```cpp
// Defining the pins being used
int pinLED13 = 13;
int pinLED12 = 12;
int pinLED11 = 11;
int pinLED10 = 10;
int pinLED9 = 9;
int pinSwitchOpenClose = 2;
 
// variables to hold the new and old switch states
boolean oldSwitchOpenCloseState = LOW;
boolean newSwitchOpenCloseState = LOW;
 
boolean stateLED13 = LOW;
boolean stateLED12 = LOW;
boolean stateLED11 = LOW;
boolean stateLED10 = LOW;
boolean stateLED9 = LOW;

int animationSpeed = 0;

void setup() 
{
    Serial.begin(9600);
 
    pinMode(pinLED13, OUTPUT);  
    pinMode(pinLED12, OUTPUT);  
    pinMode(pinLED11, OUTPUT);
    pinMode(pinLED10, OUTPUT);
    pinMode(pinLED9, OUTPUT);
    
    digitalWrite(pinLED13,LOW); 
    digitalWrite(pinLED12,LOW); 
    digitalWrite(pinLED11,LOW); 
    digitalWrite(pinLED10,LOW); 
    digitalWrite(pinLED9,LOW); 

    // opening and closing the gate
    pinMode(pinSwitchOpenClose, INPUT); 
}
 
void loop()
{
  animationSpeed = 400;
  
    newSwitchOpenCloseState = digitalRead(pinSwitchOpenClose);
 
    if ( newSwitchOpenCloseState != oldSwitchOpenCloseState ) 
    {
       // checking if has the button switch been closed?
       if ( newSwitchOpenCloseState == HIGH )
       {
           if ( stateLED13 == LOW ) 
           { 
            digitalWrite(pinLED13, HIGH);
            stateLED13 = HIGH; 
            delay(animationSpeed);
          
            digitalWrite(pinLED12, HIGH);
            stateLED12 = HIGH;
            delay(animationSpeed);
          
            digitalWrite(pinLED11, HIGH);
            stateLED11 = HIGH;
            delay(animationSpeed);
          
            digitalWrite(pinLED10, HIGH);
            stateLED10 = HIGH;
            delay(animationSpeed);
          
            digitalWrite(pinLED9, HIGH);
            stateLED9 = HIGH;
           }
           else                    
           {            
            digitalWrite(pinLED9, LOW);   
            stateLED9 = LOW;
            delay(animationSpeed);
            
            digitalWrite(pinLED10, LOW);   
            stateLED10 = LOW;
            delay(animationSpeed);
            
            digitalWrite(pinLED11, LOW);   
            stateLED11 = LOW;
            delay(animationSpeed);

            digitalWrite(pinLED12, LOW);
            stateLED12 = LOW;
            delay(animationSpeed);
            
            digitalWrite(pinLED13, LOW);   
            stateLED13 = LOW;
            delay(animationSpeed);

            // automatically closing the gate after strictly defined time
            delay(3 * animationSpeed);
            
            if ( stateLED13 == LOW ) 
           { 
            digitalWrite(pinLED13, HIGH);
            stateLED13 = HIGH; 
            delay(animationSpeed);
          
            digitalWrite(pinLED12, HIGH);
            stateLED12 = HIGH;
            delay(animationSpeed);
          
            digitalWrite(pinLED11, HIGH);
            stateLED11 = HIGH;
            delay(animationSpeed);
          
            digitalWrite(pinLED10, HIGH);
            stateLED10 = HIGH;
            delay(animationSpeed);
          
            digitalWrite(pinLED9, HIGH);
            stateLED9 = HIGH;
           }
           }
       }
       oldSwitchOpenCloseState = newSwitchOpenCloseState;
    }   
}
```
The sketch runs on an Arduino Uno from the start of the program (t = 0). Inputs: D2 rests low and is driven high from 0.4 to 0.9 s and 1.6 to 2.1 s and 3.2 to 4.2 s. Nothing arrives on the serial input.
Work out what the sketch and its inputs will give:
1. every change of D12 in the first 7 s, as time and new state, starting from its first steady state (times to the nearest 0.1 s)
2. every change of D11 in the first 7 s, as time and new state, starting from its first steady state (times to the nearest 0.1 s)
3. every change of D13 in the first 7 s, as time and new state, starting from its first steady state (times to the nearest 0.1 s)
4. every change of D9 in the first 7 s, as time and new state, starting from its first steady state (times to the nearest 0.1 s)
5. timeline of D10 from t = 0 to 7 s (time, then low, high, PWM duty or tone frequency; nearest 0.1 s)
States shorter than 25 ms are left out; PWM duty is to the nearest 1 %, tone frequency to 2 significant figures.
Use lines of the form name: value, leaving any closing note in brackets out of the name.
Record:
every change of D12 in the first 7 s, as time and new state, starting from its first steady state: 0 s low; 0.8 s high; 4.4 s low; 6.8 s high
every change of D11 in the first 7 s, as time and new state, starting from its first steady state: 0 s low; 1.2 s high; 4 s low
every change of D13 in the first 7 s, as time and new state, starting from its first steady state: 0 s low; 0.4 s high; 4.8 s low; 6.4 s high
every change of D9 in the first 7 s, as time and new state, starting from its first steady state: 0 s low; 2 s high; 3.2 s low
timeline of D10 from t = 0 to 7 s: 0 s low; 1.6 s high; 3.6 s low
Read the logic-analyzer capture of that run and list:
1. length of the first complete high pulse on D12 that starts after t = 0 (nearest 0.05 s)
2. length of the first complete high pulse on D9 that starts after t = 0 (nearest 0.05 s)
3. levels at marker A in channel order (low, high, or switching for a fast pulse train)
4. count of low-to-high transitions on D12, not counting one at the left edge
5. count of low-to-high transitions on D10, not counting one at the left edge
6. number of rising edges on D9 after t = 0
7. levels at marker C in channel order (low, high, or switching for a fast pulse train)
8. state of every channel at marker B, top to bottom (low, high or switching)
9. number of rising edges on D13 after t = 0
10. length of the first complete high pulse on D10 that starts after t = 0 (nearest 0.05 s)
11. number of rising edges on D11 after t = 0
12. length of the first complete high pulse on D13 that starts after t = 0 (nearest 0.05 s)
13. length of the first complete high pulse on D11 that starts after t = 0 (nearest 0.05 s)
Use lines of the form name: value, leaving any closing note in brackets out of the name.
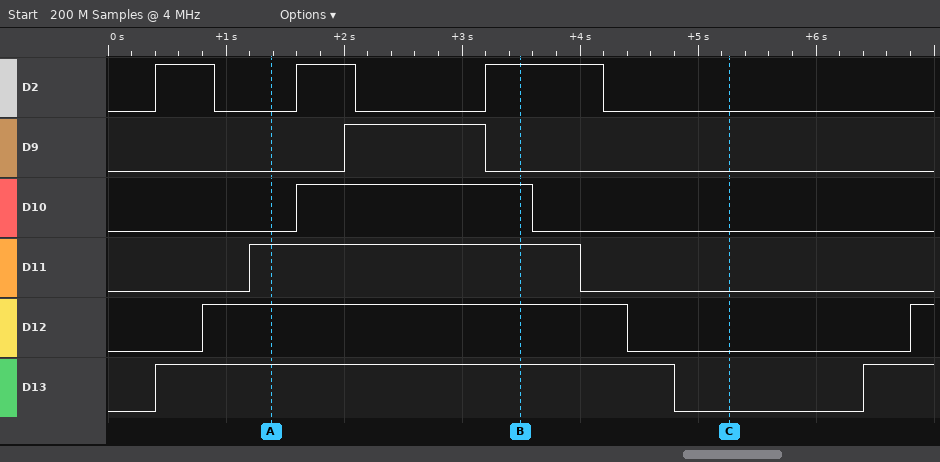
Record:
length of the first complete high pulse on D12 that starts after t = 0: 3.60 s
length of the first complete high pulse on D9 that starts after t = 0: 1.20 s
levels at marker A in channel order: D2 low, D9 low, D10 low, D11 high, D12 high, D13 high
count of low-to-high transitions on D12, not counting one at the left edge: 2
count of low-to-high transitions on D10, not counting one at the left edge: 1
number of rising edges on D9 after t = 0: 1
levels at marker C in channel order: D2 low, D9 low, D10 low, D11 low, D12 low, D13 low
state of every channel at marker B, top to bottom: D2 high, D9 low, D10 high, D11 high, D12 high, D13 high
number of rising edges on D13 after t = 0: 2
length of the first complete high pulse on D10 that starts after t = 0: 2.00 s
number of rising edges on D11 after t = 0: 1
length of the first complete high pulse on D13 that starts after t = 0: 4.40 s
length of the first complete high pulse on D11 that starts after t = 0: 2.80 s
